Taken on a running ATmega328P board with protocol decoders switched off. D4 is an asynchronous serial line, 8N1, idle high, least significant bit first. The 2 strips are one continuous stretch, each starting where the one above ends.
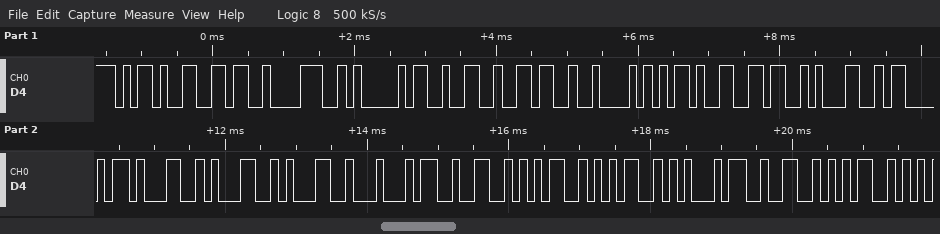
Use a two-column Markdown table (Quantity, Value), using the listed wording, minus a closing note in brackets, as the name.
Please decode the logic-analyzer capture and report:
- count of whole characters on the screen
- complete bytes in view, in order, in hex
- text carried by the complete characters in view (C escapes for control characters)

| Quantity | Value |
|---|---|
| count of whole characters on the screen | 21 |
| complete bytes in view, in order, in hex | 2D 36 38 41 32 36 42 2D 36 31 43 31 31 31 44 32 35 35 45 32 35 |
| text carried by the complete characters in view | "-68A26B-61C111D255E25" |
